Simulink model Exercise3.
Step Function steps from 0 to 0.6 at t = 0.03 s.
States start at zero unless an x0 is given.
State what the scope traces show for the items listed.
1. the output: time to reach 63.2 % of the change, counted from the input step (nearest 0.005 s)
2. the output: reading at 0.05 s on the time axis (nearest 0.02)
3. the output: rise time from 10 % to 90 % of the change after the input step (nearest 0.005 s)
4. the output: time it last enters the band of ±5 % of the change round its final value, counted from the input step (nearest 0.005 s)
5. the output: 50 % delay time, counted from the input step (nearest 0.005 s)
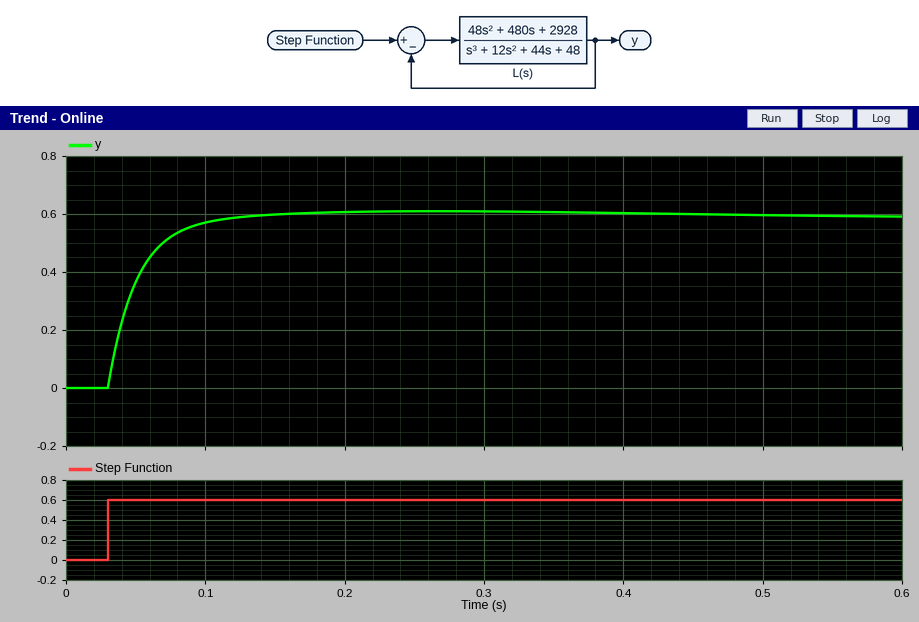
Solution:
0.020 s
0.36
0.045 s
0.065 s
0.015 s
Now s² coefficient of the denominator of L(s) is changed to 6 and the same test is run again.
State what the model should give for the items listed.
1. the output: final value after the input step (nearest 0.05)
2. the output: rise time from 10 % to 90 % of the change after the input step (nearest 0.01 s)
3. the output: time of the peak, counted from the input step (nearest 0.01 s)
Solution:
0.60
0.04 s
0.10 s
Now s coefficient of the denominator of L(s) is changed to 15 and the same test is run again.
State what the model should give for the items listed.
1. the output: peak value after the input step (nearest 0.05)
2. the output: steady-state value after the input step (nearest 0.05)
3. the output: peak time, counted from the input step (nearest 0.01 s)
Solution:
0.65
0.60
0.22 s
